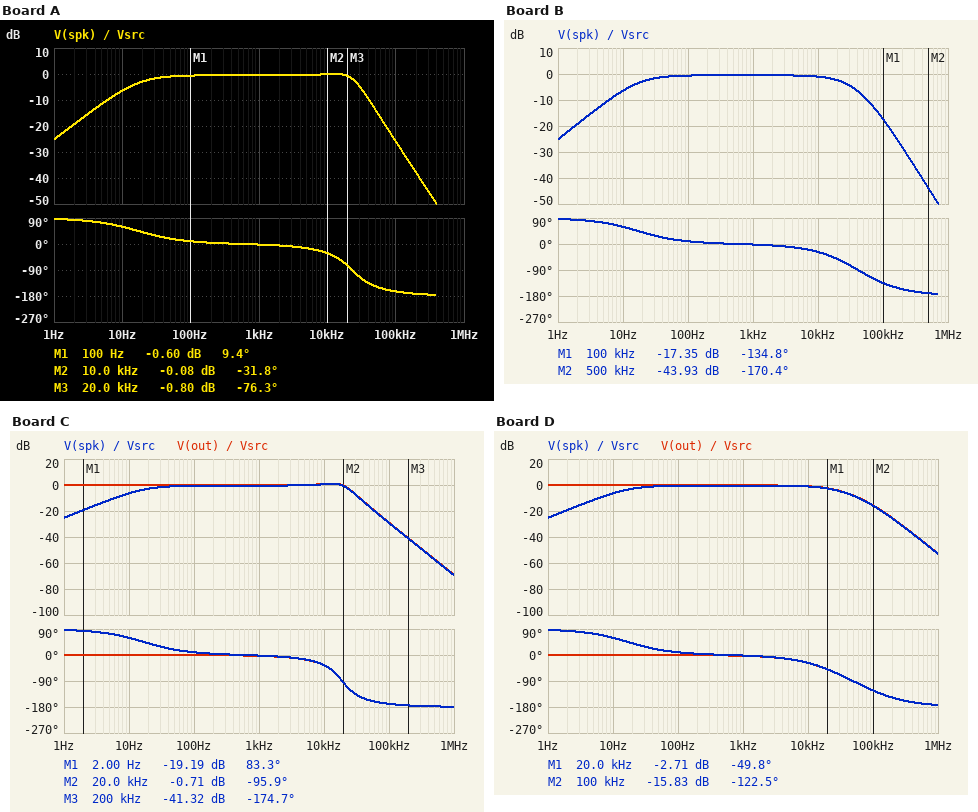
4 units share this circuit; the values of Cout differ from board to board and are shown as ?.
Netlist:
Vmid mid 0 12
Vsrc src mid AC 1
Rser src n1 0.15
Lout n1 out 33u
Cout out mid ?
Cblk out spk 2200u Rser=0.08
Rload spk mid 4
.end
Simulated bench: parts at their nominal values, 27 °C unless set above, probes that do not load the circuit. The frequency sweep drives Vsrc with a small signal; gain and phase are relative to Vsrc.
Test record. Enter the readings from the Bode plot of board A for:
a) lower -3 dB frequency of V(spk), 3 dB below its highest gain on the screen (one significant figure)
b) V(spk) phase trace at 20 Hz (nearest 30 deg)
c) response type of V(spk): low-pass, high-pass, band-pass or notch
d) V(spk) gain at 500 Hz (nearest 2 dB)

20 Hz
30 deg
band-pass
0 dB
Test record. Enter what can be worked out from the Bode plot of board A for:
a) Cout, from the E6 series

1.5 µF
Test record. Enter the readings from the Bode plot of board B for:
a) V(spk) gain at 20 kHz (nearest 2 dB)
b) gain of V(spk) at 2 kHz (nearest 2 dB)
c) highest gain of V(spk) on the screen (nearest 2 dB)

-2 dB
0 dB
0 dB
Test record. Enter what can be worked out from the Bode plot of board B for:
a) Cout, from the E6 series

470 nF
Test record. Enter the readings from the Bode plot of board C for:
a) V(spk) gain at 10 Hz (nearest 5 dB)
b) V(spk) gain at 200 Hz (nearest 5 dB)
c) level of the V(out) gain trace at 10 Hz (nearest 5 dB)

-5 dB
0 dB
0 dB
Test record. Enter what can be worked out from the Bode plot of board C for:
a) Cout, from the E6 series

2.2 µF
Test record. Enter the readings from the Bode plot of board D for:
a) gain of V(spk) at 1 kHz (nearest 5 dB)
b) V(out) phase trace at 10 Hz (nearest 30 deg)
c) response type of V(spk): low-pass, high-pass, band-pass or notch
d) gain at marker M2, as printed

0 dB
0 deg
band-pass
-15.83 dB
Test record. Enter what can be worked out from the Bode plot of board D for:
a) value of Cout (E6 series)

330 nF
